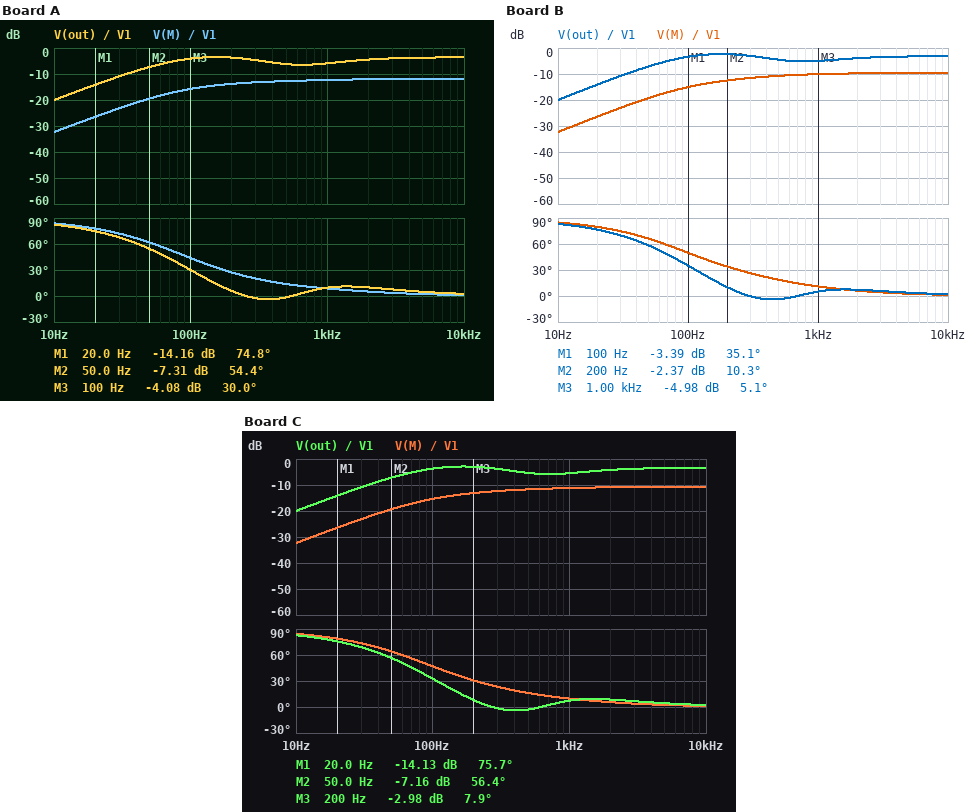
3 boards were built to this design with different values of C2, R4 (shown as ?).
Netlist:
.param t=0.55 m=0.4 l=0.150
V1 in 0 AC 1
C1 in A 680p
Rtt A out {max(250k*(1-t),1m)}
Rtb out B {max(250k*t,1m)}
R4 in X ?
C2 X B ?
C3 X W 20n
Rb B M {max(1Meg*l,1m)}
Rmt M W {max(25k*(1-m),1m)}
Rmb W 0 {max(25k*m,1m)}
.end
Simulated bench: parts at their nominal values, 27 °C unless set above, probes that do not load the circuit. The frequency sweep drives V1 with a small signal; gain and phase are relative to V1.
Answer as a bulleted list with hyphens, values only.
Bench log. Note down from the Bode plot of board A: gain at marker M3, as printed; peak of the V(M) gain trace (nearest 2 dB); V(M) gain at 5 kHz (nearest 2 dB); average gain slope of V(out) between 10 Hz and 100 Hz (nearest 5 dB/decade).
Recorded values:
- -4.08 dB
- -12 dB
- -12 dB
- 15 dB/decade
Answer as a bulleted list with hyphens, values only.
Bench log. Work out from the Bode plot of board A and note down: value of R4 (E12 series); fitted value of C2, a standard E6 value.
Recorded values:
- 33 kΩ
- 6.8 nF
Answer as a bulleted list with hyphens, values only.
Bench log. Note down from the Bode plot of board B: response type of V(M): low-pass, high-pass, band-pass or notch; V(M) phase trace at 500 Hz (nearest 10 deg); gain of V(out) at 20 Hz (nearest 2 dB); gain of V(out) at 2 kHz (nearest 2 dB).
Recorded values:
- high-pass
- 20 deg
- -14 dB
- -4 dB
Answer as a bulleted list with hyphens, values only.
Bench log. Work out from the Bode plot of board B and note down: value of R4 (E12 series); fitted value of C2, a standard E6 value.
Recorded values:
- 22 kΩ
- 6.8 nF
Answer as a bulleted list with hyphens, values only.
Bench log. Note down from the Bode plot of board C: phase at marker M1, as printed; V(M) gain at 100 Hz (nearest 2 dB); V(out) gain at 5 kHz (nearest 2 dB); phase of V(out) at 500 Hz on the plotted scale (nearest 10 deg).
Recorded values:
- 75.7 deg
- -16 dB
- -4 dB
- 0 deg
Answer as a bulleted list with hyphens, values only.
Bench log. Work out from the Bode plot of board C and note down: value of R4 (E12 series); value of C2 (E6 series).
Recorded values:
- 27 kΩ
- 6.8 nF
